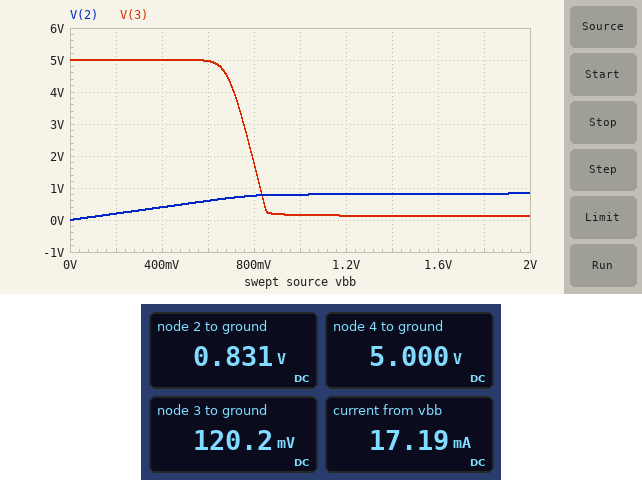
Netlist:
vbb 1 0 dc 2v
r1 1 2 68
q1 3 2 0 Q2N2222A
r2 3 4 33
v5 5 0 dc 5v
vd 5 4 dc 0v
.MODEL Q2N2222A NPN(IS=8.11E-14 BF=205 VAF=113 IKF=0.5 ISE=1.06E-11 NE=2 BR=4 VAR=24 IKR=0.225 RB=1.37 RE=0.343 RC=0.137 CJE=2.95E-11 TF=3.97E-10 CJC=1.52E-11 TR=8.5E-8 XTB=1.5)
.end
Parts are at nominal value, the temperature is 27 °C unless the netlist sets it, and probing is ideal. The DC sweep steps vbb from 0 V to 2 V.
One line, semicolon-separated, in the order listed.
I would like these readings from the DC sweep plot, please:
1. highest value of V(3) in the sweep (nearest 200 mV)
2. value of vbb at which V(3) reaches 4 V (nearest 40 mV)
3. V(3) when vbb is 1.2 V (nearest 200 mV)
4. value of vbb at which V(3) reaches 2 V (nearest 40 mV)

5.0 V; 720 mV; 200 mV; 800 mV
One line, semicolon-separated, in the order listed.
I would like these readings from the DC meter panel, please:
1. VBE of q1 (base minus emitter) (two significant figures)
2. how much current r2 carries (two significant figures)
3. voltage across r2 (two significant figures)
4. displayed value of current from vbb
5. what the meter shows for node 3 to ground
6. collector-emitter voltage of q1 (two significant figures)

830 mV; 150 mA; 4.9 V; 17.19 mA; 120.2 mV; 120 mV
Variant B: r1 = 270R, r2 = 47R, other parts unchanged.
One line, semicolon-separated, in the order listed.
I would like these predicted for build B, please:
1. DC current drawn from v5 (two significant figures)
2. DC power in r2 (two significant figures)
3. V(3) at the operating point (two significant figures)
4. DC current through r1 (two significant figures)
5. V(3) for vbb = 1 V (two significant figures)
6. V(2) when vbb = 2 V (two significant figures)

100 mA; 510 mW; 110 mV; 4.5 mA; 180 mV; 780 mV
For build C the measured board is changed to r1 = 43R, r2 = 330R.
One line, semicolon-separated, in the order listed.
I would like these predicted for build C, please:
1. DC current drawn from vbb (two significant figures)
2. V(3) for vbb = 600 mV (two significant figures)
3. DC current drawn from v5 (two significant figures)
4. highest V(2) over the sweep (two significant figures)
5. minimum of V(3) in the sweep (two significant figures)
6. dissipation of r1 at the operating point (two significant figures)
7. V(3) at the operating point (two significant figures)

28 mA; 4.7 V; 15 mA; 790 mV; 26 mV; 34 mW; 29 mV
